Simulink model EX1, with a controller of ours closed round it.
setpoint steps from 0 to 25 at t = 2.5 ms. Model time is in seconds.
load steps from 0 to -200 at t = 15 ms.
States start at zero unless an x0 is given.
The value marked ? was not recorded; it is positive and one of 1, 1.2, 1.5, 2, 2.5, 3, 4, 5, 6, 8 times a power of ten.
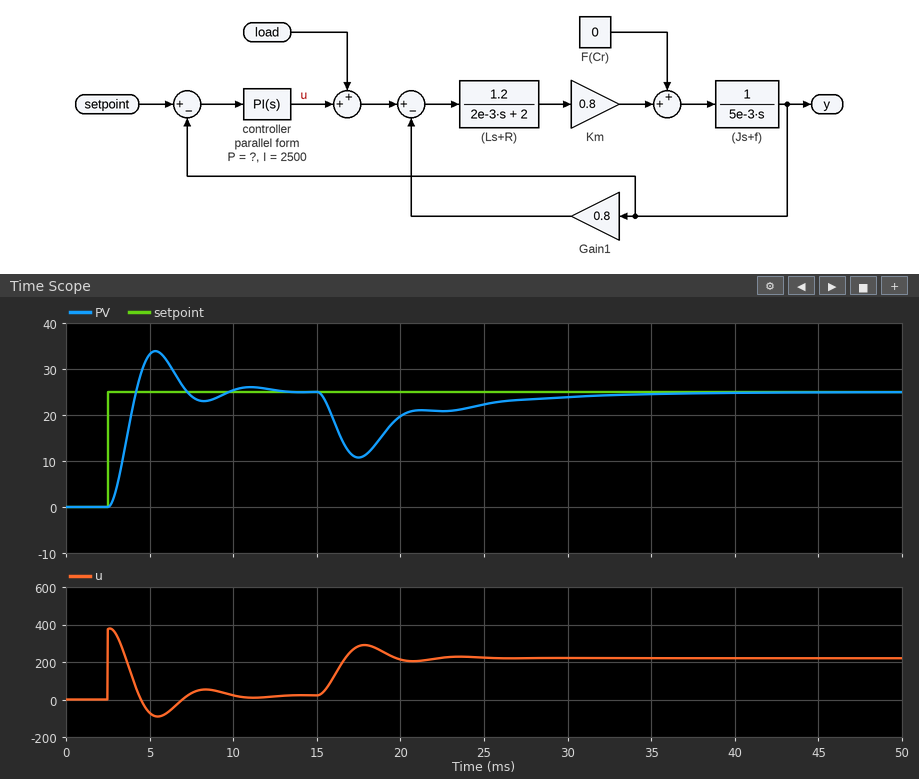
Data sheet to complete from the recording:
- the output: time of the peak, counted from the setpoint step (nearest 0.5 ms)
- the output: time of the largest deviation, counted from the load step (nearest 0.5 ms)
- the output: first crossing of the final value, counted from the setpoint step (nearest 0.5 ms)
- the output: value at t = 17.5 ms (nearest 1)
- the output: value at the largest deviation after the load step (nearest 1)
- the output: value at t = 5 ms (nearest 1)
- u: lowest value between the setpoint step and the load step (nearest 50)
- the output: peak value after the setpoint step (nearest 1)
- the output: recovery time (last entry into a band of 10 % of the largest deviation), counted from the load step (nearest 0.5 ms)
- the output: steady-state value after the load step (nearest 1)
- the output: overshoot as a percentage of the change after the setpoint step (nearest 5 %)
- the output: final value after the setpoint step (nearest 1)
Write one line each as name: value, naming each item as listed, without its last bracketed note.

the output: time of the peak, counted from the setpoint step: 3.0 ms
the output: time of the largest deviation, counted from the load step: 2.5 ms
the output: first crossing of the final value, counted from the setpoint step: 1.5 ms
the output: value at t = 17.5 ms: 11
the output: value at the largest deviation after the load step: 11
the output: value at t = 5 ms: 33
u: lowest value between the setpoint step and the load step: -100
the output: peak value after the setpoint step: 34
the output: recovery time (last entry into a band of 10 % of the largest deviation), counted from the load step: 13.5 ms
the output: steady-state value after the load step: 25
the output: overshoot as a percentage of the change after the setpoint step: 35 %
the output: final value after the setpoint step: 25
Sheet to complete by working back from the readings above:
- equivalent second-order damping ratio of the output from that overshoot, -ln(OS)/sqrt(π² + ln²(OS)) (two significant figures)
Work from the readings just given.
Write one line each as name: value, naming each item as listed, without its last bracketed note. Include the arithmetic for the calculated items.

equivalent second-order damping ratio of the output from that overshoot, -ln(OS)/sqrt(π² + ln²(OS)): ln(0.35) = -1.050; 1.050 / sqrt(9.870 + 1.102) = 0.32
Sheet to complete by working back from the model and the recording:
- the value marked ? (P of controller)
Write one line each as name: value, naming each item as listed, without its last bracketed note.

the value marked ?: 15
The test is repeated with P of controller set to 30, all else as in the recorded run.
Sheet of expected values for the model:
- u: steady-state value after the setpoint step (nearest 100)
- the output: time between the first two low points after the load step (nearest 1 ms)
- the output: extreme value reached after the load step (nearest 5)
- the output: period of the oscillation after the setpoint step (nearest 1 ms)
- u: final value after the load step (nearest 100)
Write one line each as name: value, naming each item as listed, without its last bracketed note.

u: steady-state value after the setpoint step: 0
the output: time between the first two low points after the load step: 4 ms
the output: extreme value reached after the load step: 15
the output: period of the oscillation after the setpoint step: 4 ms
u: final value after the load step: 200
